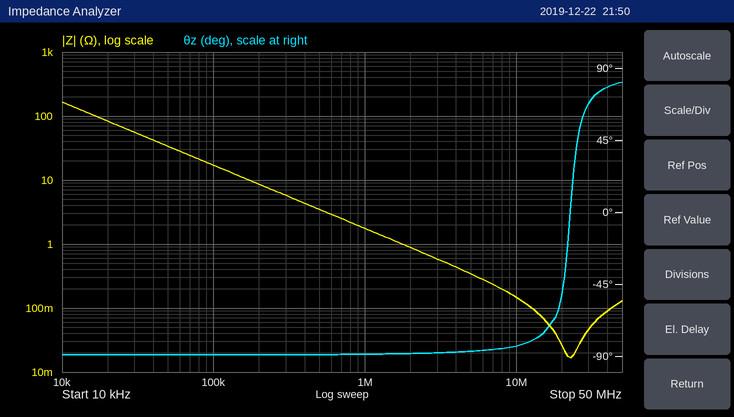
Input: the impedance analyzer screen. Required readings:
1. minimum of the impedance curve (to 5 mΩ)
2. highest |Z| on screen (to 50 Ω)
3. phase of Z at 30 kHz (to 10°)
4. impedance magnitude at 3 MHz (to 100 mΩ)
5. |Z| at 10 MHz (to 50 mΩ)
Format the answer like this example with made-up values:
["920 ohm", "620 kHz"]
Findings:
["15 mΩ", "150 Ω", "-90°", "600 mΩ", "150 mΩ"]
